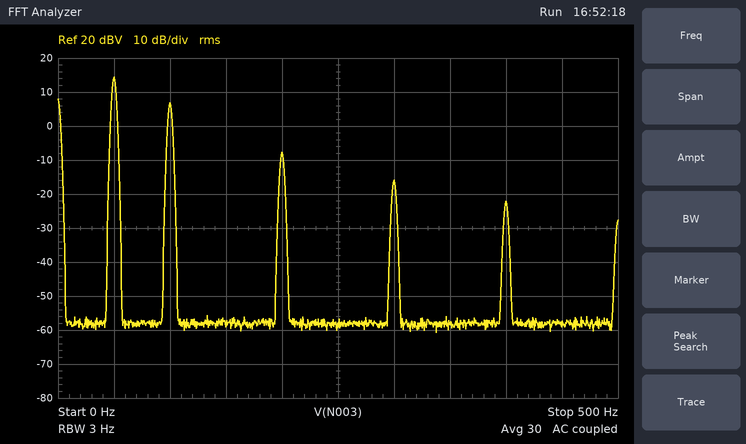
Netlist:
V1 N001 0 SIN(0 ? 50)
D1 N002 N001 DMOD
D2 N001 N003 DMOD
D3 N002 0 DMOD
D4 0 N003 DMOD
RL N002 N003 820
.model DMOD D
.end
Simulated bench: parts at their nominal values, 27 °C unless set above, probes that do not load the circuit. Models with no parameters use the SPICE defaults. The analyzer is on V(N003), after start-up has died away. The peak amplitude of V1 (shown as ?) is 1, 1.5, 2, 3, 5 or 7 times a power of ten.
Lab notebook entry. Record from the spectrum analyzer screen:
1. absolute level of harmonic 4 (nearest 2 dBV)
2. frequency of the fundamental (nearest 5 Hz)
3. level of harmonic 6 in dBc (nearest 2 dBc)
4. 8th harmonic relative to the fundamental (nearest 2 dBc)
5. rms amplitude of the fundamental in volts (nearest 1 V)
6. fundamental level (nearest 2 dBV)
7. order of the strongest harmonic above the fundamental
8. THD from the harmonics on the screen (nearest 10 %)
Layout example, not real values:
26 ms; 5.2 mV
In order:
-8 dBV; 50 Hz; -30 dBc; -36 dBc; 5 V; 14 dBV; 2; 40 %
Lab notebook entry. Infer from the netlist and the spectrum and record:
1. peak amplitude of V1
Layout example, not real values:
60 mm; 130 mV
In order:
15 V
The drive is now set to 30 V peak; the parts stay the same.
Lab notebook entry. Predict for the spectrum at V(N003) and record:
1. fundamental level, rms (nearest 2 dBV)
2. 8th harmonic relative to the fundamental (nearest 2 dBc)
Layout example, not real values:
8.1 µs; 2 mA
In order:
20 dBV; -34 dBc
